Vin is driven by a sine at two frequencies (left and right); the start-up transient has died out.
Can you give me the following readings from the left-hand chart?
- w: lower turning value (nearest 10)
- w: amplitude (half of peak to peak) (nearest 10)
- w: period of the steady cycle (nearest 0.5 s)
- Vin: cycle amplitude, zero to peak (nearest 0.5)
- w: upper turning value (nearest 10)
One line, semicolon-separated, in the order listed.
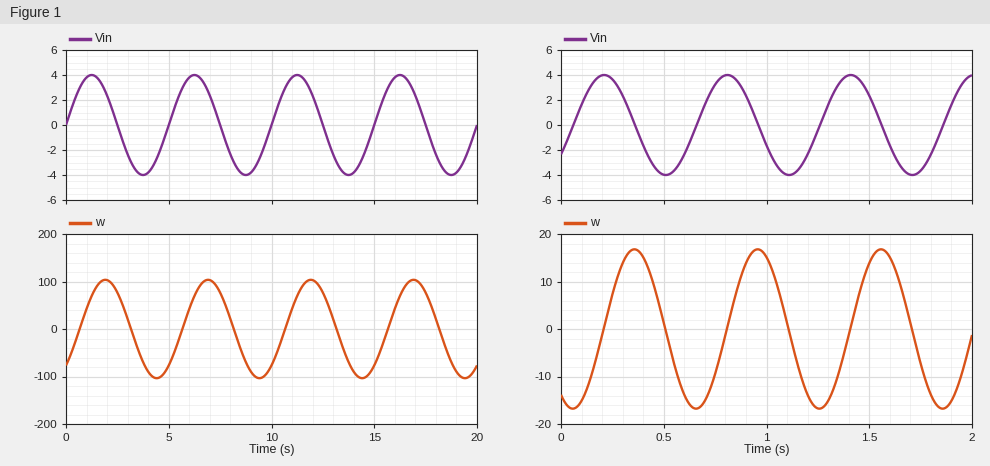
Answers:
-100; 100; 5.0 s; 4.0; 100
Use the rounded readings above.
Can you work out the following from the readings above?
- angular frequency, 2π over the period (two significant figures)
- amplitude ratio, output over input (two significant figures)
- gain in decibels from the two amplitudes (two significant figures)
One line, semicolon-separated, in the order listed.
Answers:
1.3 rad/s; 25; 28 dB
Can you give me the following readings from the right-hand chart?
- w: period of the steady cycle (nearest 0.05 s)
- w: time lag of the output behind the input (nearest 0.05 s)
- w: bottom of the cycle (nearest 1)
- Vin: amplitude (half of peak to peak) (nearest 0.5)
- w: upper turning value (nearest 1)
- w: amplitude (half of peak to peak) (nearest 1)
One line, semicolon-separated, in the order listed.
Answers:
0.60 s; 0.15 s; -17; 4.0; 17; 17
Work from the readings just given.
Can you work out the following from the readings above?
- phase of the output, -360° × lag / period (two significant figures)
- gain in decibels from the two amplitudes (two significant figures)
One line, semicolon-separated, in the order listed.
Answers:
-90°; 13 dB
